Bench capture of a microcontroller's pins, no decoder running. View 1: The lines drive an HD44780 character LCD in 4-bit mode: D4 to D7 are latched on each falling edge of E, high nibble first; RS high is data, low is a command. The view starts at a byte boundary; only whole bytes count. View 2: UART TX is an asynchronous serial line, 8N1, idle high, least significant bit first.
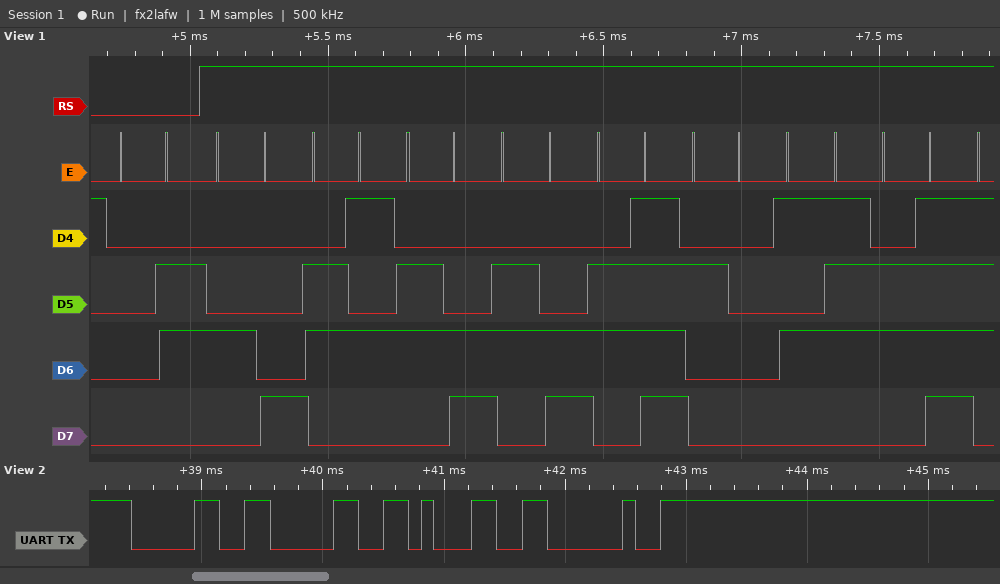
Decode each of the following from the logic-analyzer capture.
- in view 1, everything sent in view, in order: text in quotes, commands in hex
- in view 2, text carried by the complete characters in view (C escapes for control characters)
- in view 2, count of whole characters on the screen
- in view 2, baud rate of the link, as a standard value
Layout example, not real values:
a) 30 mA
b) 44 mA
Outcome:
a) 0x06 "Hello Wo"
b) "001 "
c) 4
d) 9600 baud
